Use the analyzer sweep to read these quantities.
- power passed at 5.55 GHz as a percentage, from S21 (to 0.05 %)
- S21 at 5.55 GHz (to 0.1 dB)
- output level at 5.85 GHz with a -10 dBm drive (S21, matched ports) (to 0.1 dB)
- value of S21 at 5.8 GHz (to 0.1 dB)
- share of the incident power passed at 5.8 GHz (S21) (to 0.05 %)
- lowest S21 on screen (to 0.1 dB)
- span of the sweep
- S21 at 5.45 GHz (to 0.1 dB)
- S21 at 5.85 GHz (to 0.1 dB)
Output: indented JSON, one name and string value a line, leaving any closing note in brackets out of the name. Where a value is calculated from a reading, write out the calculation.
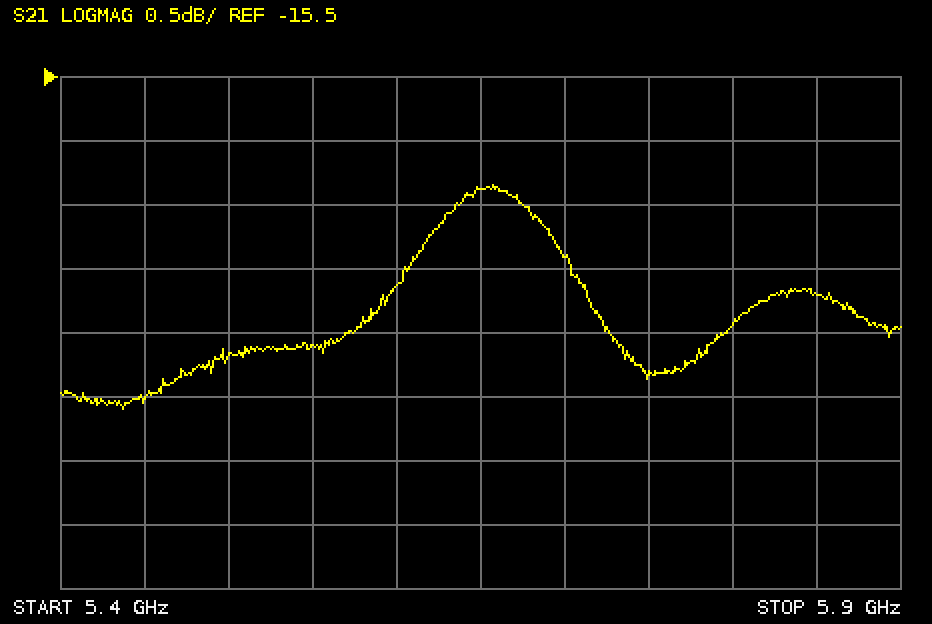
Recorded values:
{
  "power passed at 5.55 GHz as a percentage, from S21": "10^(-17.6/10) ≈ 1.74 %, so 1.75 % to the nearest 0.05 %",
  "S21 at 5.55 GHz": "-17.6 dB",
  "output level at 5.85 GHz with a -10 dBm drive (S21, matched ports)": "-10 dBm + (-17.2 dB) = -27.2 dBm",
  "value of S21 at 5.8 GHz": "-17.4 dB",
  "share of the incident power passed at 5.8 GHz (S21)": "10^(-17.4/10) ≈ 1.82 %, so 1.80 % to the nearest 0.05 %",
  "lowest S21 on screen": "-18.1 dB",
  "span of the sweep": "500 MHz",
  "S21 at 5.45 GHz": "-18.0 dB",
  "S21 at 5.85 GHz": "-17.2 dB"
}
